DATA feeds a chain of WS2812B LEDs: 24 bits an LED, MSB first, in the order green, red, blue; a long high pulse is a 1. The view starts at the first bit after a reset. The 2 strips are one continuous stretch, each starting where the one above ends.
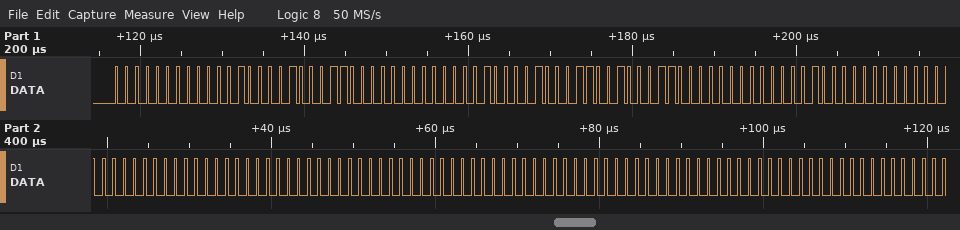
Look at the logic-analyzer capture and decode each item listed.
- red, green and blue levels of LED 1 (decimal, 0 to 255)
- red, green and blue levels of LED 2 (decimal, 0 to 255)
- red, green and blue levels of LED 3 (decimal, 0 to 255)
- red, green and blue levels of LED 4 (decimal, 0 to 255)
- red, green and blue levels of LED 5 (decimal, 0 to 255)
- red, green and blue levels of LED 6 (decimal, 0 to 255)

8, 0, 70
8, 0, 70
0, 70, 8
0, 0, 0
0, 0, 0
0, 0, 0
